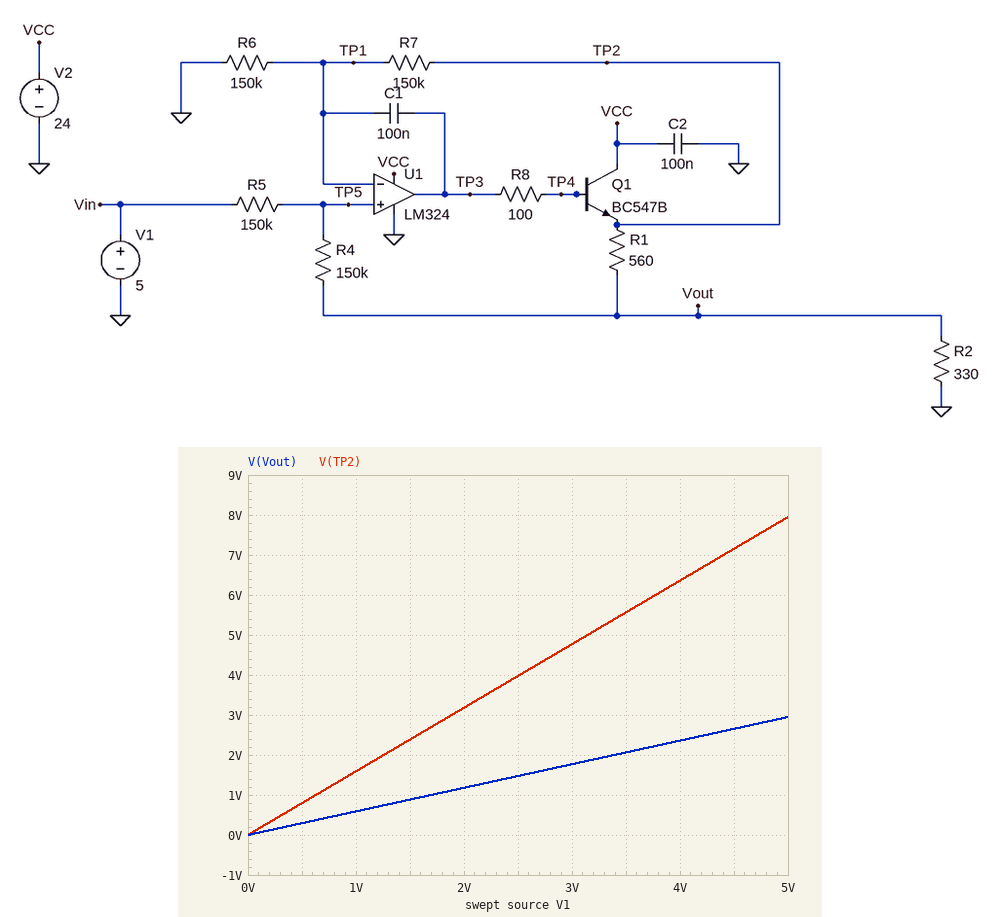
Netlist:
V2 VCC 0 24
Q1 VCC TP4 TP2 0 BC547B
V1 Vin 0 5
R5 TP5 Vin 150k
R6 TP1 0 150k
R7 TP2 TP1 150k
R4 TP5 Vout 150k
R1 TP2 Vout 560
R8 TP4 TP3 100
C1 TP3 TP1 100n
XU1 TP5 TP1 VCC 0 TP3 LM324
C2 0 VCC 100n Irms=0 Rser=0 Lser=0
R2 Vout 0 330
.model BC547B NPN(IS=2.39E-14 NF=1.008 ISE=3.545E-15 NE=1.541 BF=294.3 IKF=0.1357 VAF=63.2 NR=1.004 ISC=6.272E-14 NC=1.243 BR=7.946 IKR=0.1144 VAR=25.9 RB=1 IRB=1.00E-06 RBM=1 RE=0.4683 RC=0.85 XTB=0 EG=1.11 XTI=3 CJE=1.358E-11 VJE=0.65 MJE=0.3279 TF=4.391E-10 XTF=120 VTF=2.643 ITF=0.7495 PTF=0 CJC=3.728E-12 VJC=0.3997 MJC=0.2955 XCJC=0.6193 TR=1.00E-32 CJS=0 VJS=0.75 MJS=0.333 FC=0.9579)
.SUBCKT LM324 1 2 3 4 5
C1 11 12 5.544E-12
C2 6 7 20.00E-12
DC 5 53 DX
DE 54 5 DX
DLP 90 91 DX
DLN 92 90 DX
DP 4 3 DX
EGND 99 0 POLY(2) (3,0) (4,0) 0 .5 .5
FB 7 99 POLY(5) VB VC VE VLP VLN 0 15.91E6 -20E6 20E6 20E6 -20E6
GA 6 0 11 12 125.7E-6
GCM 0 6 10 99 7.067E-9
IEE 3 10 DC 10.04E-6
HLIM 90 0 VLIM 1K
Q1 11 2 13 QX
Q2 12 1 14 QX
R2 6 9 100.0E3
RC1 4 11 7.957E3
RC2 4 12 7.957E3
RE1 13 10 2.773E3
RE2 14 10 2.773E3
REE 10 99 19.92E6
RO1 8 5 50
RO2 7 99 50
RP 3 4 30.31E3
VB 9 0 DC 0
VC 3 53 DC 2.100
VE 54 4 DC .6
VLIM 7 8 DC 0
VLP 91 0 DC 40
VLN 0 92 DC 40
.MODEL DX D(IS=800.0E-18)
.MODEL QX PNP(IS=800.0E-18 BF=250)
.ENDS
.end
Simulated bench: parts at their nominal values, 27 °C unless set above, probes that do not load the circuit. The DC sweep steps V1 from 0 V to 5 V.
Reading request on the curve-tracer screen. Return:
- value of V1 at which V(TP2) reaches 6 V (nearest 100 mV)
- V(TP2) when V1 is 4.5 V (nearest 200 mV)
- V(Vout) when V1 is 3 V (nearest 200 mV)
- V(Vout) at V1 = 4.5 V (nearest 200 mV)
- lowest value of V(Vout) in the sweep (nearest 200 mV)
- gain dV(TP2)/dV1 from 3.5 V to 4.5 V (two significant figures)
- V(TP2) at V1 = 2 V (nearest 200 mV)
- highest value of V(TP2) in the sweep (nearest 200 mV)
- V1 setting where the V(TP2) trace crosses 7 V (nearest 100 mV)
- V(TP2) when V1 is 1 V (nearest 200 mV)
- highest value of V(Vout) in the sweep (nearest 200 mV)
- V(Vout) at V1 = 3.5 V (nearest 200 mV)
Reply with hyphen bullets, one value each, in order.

- 3.8 V
- 7.2 V
- 1.8 V
- 2.6 V
- 0 V
- 1.6 V/V
- 3.2 V
- 8.0 V
- 4.4 V
- 1.6 V
- 3.0 V
- 2.0 V
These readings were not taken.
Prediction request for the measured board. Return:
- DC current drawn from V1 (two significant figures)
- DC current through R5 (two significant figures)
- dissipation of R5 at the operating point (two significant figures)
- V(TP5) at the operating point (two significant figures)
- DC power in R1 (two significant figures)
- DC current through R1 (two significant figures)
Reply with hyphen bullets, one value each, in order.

- 6.8 µA
- 6.8 µA
- 7.0 µW
- 4.0 V
- 45 mW
- 8.9 mA
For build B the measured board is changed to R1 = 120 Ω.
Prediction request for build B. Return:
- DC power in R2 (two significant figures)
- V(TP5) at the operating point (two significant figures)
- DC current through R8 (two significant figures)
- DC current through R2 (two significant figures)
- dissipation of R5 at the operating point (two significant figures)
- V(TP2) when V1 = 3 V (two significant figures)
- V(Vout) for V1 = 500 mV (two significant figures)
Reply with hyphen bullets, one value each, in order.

- 570 mW
- 9.4 V
- 180 µA
- 42 mA
- 130 µW
- 11 V
- 1.4 V
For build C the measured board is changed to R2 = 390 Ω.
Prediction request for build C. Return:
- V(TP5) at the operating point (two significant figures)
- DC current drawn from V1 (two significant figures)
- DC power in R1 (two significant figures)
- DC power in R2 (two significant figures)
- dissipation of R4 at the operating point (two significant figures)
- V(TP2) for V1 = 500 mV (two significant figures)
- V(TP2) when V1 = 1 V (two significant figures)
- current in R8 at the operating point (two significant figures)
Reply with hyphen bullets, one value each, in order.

- 4.2 V
- 5.0 µA
- 45 mW
- 31 mW
- 3.8 µW
- 850 mV
- 1.7 V
- 27 µA
